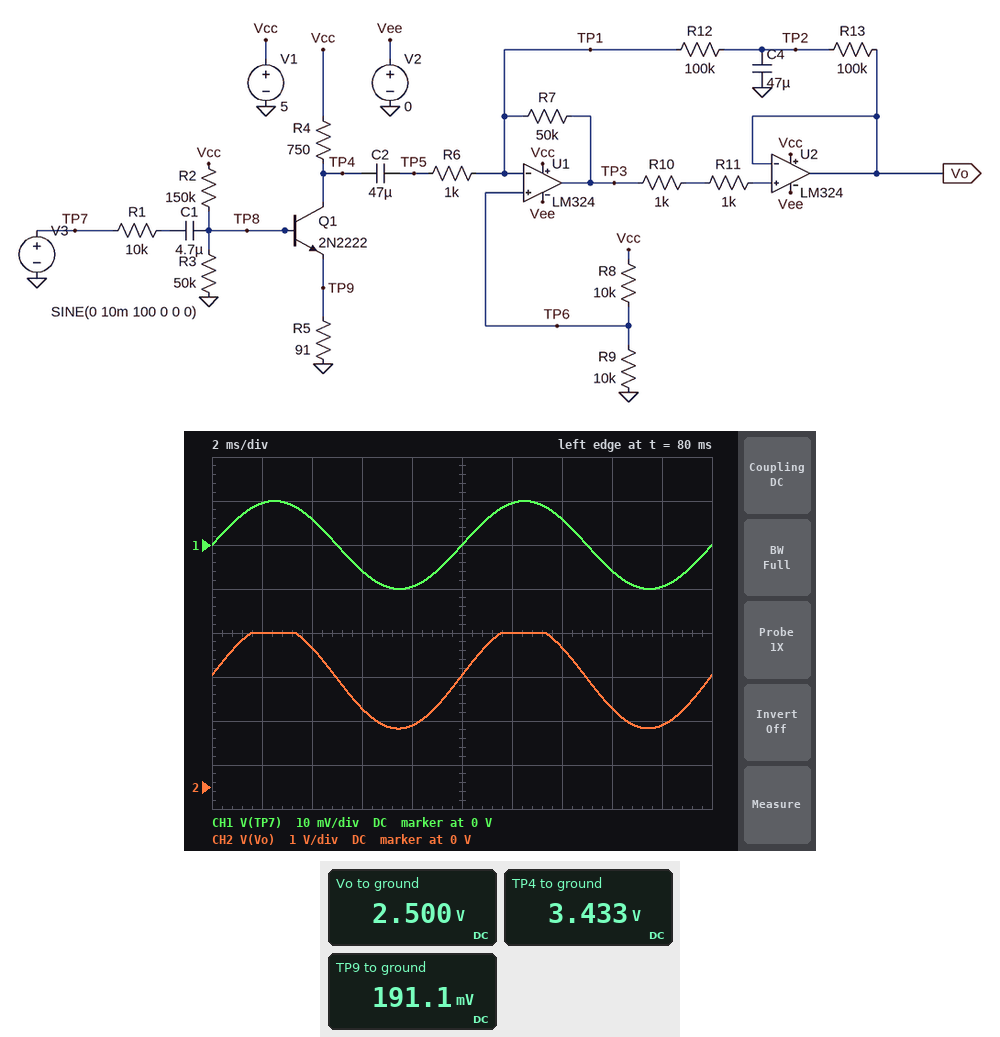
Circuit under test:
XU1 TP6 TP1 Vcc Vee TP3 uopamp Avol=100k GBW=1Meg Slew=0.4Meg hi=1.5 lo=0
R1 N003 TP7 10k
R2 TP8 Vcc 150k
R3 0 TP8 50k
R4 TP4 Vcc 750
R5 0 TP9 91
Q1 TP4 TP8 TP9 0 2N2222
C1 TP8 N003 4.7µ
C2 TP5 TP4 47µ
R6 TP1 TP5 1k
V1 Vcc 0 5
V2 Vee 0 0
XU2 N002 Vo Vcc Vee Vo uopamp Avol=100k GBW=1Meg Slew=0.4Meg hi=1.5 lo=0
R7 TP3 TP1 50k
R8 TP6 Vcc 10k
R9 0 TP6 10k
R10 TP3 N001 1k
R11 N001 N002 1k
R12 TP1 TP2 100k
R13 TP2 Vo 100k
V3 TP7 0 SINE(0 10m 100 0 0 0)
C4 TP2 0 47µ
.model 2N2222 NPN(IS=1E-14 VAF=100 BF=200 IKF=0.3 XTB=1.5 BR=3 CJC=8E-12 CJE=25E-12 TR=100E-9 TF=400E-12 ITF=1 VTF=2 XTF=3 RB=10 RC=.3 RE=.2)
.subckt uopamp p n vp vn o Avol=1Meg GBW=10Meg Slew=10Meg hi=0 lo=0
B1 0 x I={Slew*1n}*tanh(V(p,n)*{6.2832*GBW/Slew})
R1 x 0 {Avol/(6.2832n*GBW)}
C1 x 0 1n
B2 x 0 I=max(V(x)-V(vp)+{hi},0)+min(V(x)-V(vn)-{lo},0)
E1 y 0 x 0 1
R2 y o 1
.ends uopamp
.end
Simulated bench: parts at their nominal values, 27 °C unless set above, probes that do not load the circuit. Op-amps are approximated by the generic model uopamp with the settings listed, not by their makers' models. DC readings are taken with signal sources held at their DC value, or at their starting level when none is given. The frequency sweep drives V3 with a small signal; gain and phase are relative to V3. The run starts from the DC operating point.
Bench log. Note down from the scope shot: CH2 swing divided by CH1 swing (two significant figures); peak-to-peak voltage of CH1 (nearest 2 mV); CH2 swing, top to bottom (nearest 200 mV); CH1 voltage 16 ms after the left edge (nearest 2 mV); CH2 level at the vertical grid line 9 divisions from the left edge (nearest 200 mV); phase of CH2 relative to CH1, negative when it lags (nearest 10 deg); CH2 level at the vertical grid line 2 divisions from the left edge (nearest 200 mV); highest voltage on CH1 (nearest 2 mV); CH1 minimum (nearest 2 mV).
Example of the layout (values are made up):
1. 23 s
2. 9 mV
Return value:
1. 110
2. 20 mV
3. 2.2 V
4. -6 mV
5. 1.4 V
6. 0 deg
7. 3.2 V
8. 10 mV
9. -10 mV
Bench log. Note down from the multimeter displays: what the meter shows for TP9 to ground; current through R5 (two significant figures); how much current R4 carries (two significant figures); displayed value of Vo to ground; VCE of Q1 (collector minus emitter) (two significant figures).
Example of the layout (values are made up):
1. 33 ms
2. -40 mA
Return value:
1. 191.1 mV
2. 2.1 mA
3. 2.1 mA
4. 2.500 V
5. 3.2 V
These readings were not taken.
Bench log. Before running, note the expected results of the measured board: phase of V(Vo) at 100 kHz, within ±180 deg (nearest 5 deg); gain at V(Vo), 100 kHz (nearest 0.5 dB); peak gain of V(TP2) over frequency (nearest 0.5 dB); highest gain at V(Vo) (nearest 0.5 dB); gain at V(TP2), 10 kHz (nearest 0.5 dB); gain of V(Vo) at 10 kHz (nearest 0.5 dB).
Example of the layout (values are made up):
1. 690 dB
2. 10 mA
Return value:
1. -85 deg
2. 31.5 dB
3. 1.5 dB
4. 41.5 dB
5. -68.5 dB
6. 41.0 dB
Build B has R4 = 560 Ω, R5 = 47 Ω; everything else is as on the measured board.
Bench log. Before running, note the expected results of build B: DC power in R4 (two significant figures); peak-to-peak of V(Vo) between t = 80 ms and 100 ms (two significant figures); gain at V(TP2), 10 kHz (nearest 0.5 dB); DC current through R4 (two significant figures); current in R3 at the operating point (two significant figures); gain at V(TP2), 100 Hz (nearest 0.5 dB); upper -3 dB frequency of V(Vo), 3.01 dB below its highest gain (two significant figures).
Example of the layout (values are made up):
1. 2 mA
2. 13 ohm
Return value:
1. 3.4 mW
2. 2.4 V
3. -66.5 dB
4. 2.5 mA
5. 16 µA
6. -26.0 dB
7. 30 kHz
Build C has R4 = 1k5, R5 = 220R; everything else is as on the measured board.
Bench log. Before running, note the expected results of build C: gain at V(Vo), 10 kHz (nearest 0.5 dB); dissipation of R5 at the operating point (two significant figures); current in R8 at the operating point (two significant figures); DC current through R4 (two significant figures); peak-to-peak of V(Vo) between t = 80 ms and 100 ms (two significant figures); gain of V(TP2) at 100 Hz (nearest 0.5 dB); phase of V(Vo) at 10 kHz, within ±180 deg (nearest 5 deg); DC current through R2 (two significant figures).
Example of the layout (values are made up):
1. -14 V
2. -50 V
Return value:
1. 38.5 dB
2. 460 µW
3. 250 µA
4. 1.4 mA
5. 1.7 V
6. -31.0 dB
7. -15 deg
8. 27 µA
